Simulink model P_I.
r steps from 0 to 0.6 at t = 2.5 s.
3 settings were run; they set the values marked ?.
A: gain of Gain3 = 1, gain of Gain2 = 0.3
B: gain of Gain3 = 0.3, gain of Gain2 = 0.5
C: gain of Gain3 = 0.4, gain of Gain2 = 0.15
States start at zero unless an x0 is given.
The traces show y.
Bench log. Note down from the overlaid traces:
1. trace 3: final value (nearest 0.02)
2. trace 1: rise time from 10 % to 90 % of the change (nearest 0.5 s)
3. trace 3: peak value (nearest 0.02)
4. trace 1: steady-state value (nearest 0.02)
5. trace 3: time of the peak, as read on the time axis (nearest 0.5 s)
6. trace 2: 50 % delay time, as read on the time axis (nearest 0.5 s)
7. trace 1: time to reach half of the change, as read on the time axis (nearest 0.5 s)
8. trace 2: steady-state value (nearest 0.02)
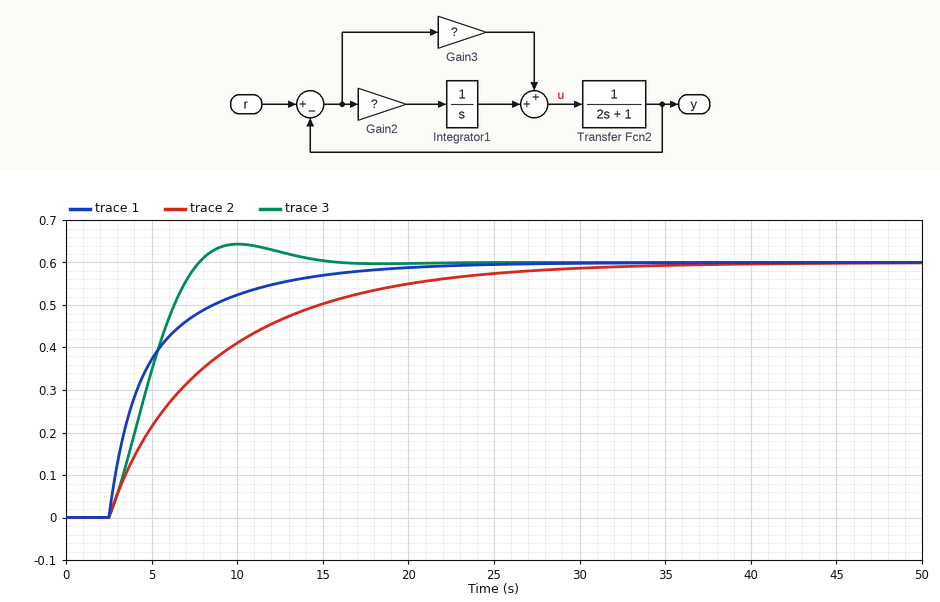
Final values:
0.60
8.5 s
0.64
0.60
10.0 s
6.5 s
4.0 s
0.60
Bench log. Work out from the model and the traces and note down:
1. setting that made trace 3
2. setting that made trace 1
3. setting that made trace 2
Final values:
B
A
C
